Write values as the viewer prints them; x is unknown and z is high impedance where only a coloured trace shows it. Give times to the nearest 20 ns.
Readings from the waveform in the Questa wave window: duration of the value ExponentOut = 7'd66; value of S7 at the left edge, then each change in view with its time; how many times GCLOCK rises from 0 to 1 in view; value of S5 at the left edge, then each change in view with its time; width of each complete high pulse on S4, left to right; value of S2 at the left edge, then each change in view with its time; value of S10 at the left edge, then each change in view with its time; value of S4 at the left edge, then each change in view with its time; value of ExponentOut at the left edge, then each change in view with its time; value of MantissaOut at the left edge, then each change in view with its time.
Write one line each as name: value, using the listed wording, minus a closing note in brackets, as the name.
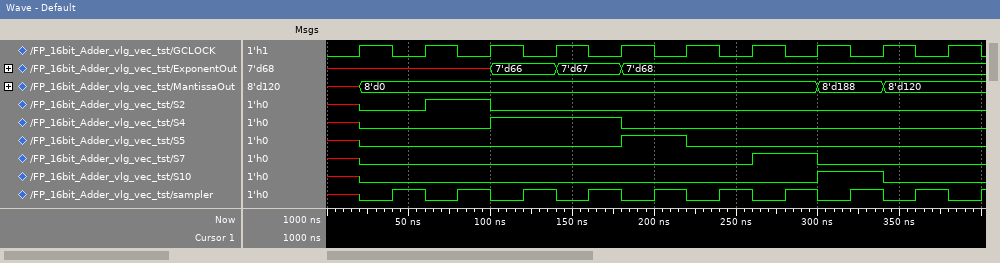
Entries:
duration of the value ExponentOut = 7'd66: 40 ns
value of S7 at the left edge, then each change in view with its time: x, 0 at 20 ns, 1 at 260 ns, 0 at 300 ns
how many times GCLOCK rises from 0 to 1 in view: 10
value of S5 at the left edge, then each change in view with its time: x, 0 at 20 ns, 1 at 180 ns, 0 at 220 ns
width of each complete high pulse on S4, left to right: 80 ns
value of S2 at the left edge, then each change in view with its time: x, 0 at 20 ns, 1 at 60 ns, 0 at 100 ns
value of S10 at the left edge, then each change in view with its time: x, 0 at 20 ns, 1 at 300 ns, 0 at 340 ns
value of S4 at the left edge, then each change in view with its time: x, 0 at 20 ns, 1 at 100 ns, 0 at 180 ns
value of ExponentOut at the left edge, then each change in view with its time: x, 7'd66 at 100 ns, 7'd67 at 140 ns, 7'd68 at 180 ns
value of MantissaOut at the left edge, then each change in view with its time: x, 8'd0 at 20 ns, 8'd188 at 300 ns, 8'd120 at 340 ns
